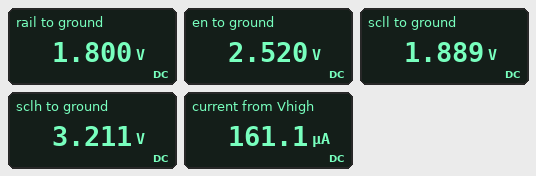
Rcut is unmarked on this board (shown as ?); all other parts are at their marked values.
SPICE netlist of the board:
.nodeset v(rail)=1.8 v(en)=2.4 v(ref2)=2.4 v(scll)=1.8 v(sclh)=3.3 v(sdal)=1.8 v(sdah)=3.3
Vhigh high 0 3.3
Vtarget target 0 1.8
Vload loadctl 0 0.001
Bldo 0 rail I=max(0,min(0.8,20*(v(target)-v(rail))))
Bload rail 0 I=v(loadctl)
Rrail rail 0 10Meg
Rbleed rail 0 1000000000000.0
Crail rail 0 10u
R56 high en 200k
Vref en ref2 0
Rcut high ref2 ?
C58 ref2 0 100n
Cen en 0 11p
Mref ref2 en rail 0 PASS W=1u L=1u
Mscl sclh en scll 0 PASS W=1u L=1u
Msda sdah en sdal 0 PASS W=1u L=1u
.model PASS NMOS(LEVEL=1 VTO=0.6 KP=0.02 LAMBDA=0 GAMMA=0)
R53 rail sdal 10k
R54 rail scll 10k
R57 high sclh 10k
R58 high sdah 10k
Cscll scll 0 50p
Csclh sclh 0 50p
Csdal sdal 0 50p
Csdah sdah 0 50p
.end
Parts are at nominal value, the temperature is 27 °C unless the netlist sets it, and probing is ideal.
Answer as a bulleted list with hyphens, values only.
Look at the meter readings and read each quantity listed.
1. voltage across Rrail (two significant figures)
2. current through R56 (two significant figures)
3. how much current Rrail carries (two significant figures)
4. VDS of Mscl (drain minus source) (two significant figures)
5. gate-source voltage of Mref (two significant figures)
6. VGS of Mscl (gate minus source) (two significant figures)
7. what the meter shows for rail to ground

- 1.8 V
- 3.9 µA
- 180 nA
- 1.3 V
- 720 mV
- 630 mV
- 1.800 V
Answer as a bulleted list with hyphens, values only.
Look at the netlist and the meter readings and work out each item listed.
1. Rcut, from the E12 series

- 5.6 kΩ
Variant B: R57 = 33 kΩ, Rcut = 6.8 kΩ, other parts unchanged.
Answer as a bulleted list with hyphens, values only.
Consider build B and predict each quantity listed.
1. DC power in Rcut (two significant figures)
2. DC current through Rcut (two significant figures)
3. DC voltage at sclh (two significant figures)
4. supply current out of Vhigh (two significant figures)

- 92 µW
- 120 µA
- 3.0 V
- 140 µA
